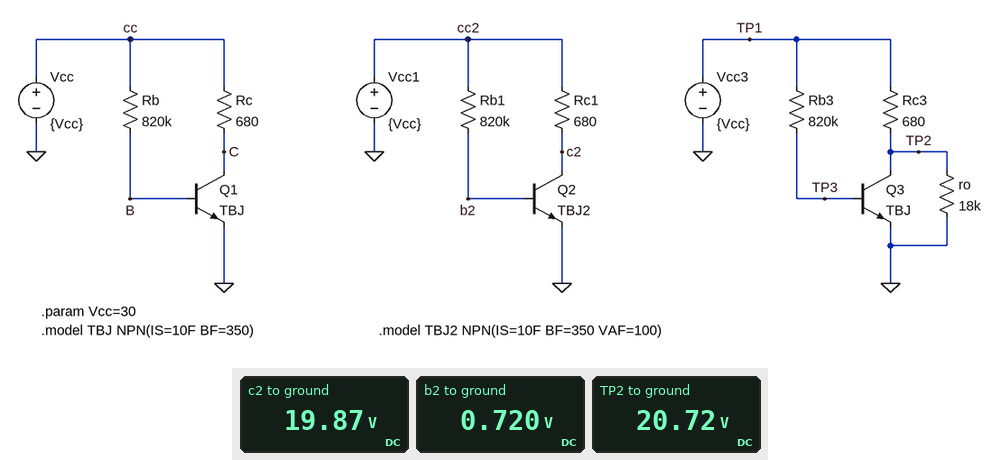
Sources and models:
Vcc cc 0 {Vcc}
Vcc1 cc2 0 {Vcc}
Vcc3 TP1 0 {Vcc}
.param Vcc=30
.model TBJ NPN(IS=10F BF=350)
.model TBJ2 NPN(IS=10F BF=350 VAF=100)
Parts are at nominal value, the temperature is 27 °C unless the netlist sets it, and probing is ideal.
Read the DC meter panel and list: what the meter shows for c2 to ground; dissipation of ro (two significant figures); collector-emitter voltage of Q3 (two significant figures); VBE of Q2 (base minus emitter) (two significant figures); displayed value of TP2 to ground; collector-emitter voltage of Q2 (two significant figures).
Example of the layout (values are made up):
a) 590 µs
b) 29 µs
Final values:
a) 19.87 V
b) 24 mW
c) 21 V
d) 720 mV
e) 20.72 V
f) 20 V
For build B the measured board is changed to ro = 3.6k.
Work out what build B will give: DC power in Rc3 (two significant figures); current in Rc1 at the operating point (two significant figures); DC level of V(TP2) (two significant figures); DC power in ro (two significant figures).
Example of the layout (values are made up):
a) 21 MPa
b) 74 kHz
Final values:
a) 210 mW
b) 15 mA
c) 18 V
d) 91 mW
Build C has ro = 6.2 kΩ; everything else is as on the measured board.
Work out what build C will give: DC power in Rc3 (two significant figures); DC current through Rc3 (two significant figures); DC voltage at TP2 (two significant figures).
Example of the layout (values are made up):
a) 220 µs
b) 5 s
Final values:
a) 170 mW
b) 16 mA
c) 19 V
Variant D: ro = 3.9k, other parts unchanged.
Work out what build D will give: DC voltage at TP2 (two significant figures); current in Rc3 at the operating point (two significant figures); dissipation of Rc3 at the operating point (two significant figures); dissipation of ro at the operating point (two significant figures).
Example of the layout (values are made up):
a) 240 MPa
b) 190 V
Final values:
a) 18 V
b) 17 mA
c) 200 mW
d) 86 mW
